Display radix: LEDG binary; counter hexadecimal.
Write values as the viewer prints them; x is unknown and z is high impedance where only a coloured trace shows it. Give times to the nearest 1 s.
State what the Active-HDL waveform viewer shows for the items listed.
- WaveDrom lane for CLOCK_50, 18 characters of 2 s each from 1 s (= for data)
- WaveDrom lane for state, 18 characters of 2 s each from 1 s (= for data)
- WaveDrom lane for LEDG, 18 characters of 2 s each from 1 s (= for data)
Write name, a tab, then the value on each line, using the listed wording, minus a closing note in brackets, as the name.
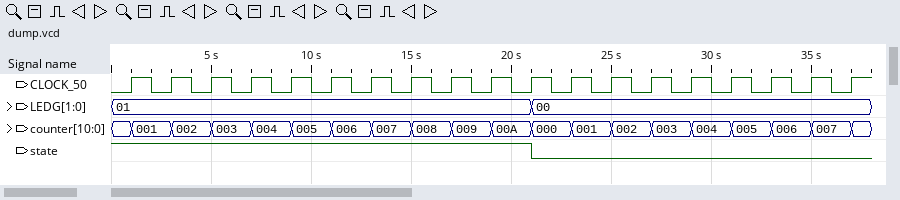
WaveDrom lane for CLOCK_50, 18 characters of 2 s each from 1 s	{name: 'CLOCK_50', wave: 'p.................'}
WaveDrom lane for state, 18 characters of 2 s each from 1 s	{name: 'state', wave: '1.........0.......'}
WaveDrom lane for LEDG, 18 characters of 2 s each from 1 s	{name: 'LEDG', wave: '=.........=.......', data: '01 00'}
